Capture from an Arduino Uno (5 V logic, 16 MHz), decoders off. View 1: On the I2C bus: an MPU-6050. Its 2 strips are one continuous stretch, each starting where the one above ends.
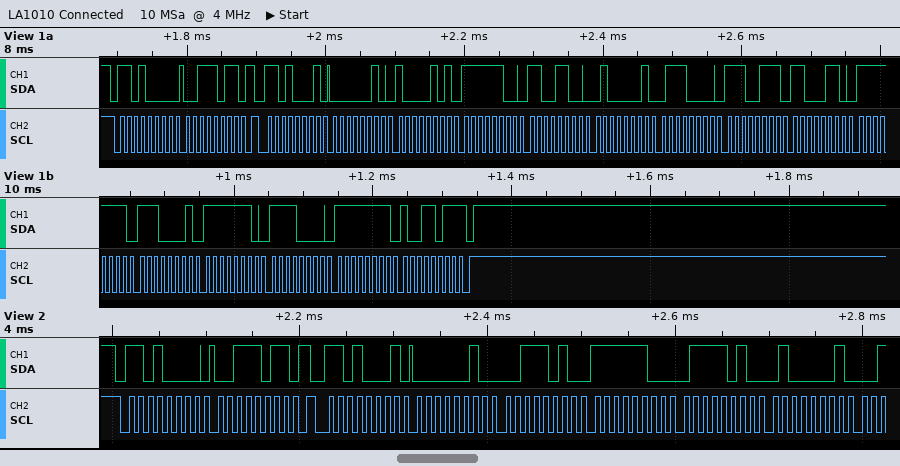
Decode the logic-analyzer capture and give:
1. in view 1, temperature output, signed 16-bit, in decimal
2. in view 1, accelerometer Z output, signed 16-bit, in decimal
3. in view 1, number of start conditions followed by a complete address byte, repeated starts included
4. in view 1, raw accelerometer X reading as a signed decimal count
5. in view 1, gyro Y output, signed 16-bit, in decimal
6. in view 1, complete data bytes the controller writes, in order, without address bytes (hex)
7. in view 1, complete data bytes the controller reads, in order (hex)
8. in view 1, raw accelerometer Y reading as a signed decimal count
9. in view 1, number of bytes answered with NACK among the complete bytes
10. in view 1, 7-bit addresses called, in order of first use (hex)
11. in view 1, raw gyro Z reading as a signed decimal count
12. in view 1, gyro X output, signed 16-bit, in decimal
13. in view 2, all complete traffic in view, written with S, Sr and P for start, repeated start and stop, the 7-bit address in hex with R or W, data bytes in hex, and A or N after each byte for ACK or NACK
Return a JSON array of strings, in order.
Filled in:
["-6202", "16752", "2", "645", "-272", "3B", "02 85 FC CC 41 70 E7 C6 FF E1 FE F0 FF 9B", "-820", "1", "0x68", "-101", "-31", "S 68W A 3B A Sr 68R A 02 A 3A A FC A 7A A 41 A"]
